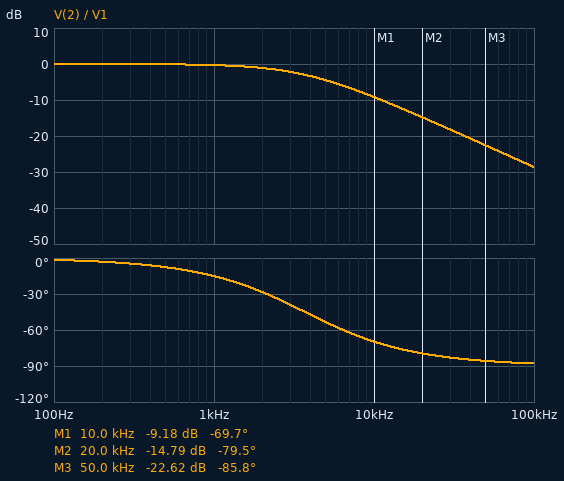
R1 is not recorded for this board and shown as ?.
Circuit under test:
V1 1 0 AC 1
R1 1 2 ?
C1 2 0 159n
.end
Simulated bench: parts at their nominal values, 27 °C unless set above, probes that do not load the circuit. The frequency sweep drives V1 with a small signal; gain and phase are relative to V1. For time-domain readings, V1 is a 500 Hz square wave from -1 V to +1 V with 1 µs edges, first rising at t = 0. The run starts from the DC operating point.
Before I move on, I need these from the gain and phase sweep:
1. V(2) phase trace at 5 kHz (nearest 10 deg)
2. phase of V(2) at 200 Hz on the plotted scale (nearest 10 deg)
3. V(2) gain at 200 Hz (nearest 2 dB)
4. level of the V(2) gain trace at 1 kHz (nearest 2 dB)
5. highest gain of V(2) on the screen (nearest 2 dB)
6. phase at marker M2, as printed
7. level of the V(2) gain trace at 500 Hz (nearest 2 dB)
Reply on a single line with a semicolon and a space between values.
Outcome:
-50 deg; 0 deg; 0 dB; 0 dB; 0 dB; -79.5 deg; 0 dB
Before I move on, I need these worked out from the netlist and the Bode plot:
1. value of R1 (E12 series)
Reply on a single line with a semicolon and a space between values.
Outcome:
270 Ω
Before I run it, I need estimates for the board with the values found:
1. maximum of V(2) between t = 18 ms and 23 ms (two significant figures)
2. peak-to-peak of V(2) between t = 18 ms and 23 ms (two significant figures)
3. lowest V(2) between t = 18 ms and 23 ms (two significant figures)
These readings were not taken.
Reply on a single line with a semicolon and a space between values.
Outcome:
1.0 V; 2.0 V; -1.0 V
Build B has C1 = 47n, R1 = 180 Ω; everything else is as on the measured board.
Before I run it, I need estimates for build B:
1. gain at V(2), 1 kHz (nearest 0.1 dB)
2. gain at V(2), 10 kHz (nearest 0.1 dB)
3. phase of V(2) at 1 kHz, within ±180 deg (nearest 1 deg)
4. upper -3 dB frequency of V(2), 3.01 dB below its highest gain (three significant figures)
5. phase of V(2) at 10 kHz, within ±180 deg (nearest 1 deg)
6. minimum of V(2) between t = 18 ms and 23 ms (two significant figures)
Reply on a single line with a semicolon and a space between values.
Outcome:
0 dB; -1.1 dB; -3 deg; 18.8 kHz; -28 deg; -1.0 V
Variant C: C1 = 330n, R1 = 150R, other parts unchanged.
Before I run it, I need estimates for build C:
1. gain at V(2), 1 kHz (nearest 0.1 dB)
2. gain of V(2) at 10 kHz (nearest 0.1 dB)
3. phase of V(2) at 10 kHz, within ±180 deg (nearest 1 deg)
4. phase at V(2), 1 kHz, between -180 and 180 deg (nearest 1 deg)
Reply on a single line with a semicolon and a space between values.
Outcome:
-0.4 dB; -10.3 dB; -72 deg; -17 deg
